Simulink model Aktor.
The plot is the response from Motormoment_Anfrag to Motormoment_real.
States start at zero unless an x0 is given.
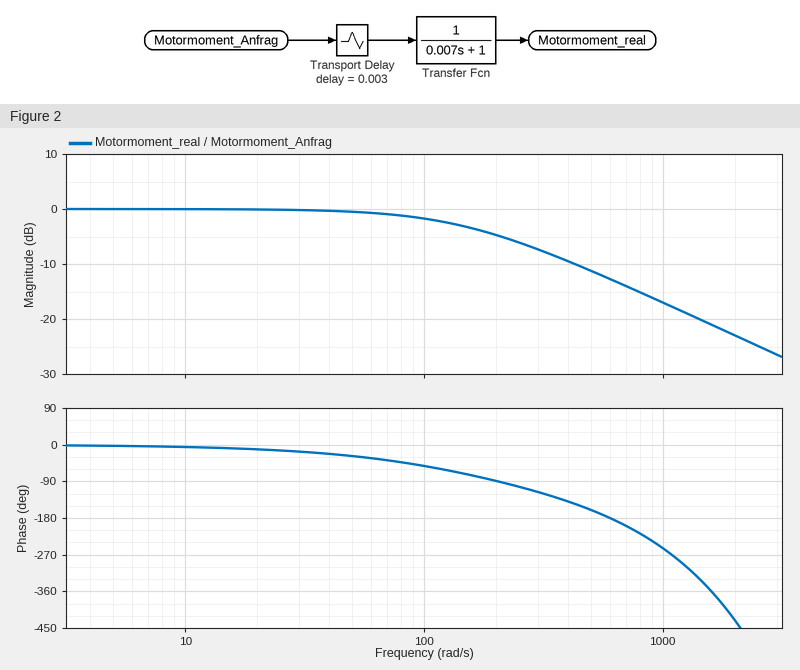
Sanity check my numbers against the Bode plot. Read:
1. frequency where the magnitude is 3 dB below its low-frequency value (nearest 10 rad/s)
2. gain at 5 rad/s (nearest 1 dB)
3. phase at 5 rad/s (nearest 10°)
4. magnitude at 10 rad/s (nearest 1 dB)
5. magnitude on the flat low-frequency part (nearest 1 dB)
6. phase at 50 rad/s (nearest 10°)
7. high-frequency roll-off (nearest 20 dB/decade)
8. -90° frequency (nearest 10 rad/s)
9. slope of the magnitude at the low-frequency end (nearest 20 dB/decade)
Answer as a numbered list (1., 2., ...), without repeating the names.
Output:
1. 140 rad/s
2. 0 dB
3. 0°
4. 0 dB
5. 0 dB
6. -30°
7. -20 dB/decade
8. 200 rad/s
9. 0 dB/decade
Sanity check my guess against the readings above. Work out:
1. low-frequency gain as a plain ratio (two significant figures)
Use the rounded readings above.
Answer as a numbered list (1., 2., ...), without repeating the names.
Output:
1. 1.0
